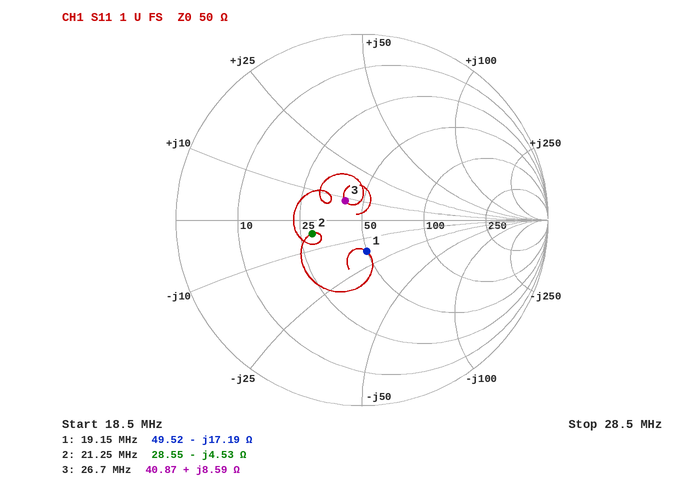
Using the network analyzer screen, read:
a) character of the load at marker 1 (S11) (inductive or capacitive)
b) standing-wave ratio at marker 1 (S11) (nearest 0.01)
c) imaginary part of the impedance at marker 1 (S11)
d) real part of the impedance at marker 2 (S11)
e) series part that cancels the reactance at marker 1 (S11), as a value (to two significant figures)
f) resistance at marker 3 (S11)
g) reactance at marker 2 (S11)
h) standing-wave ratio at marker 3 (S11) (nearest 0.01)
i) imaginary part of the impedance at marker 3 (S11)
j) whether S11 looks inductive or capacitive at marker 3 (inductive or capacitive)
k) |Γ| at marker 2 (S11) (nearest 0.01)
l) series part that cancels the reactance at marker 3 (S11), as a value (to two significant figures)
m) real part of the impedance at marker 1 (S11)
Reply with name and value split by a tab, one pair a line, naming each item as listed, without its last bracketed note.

character of the load at marker 1 (S11)	capacitive
standing-wave ratio at marker 1 (S11)	1.41
imaginary part of the impedance at marker 1	-17.19 Ω
real part of the impedance at marker 2	28.55 Ω
series part that cancels the reactance at marker 1 (S11), as a value	140 nH
resistance at marker 3	40.87 Ω
reactance at marker 2	-4.53 Ω
standing-wave ratio at marker 3 (S11)	1.32
imaginary part of the impedance at marker 3	+8.59 Ω
whether S11 looks inductive or capacitive at marker 3	inductive
|Γ| at marker 2 (S11)	0.28
series part that cancels the reactance at marker 3 (S11), as a value	690 pF
real part of the impedance at marker 1	49.52 Ω
